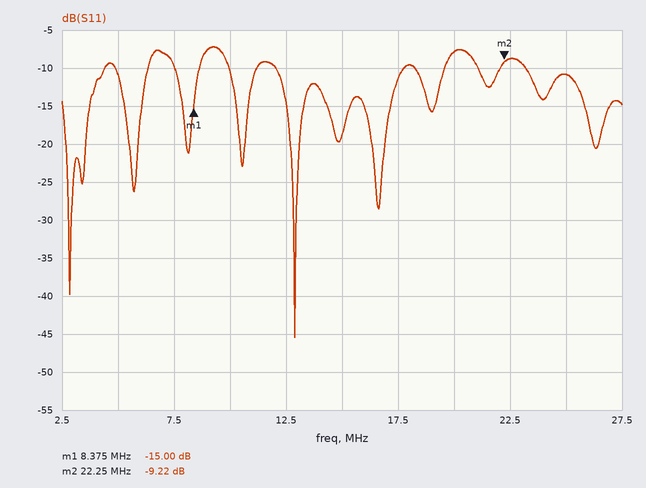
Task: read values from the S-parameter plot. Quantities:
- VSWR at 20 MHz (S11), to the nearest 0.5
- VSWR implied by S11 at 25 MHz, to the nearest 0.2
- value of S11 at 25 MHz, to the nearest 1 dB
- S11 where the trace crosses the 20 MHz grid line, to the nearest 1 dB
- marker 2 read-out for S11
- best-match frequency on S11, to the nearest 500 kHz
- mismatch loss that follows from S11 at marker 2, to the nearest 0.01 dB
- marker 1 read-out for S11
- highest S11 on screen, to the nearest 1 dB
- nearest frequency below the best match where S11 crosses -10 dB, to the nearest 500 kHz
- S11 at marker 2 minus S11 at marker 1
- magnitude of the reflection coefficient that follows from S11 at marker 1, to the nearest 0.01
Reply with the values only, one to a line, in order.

2.5
1.8
-11 dB
-8 dB
-9.22 dB
13.0 MHz
0.55 dB
-15.00 dB
-7 dB
12.0 MHz
5.78 dB
0.18
